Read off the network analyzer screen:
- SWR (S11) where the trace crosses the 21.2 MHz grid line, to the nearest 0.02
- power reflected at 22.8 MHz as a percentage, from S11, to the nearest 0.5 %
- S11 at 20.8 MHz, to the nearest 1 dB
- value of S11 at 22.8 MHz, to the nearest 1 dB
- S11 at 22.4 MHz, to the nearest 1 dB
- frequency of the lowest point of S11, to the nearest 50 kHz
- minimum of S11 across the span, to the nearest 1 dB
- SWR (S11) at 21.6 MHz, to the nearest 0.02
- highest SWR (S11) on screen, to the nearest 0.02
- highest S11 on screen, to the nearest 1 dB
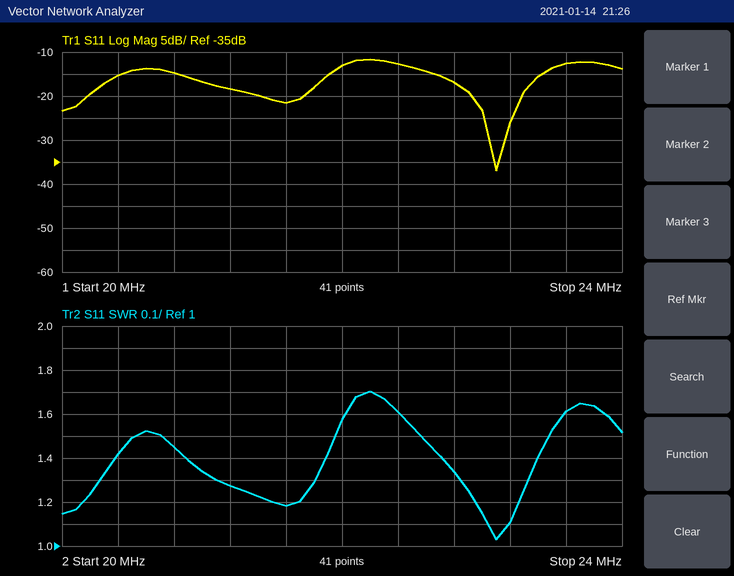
1.28
2.0 %
-15 dB
-17 dB
-13 dB
23.10 MHz
-37 dB
1.18
1.70
-12 dB
